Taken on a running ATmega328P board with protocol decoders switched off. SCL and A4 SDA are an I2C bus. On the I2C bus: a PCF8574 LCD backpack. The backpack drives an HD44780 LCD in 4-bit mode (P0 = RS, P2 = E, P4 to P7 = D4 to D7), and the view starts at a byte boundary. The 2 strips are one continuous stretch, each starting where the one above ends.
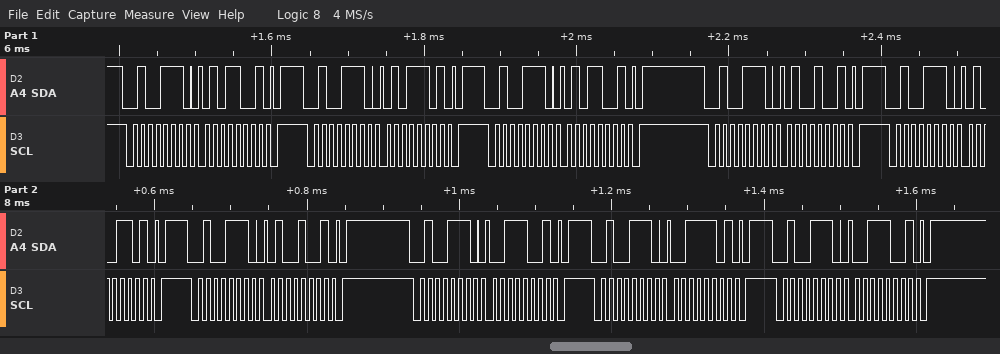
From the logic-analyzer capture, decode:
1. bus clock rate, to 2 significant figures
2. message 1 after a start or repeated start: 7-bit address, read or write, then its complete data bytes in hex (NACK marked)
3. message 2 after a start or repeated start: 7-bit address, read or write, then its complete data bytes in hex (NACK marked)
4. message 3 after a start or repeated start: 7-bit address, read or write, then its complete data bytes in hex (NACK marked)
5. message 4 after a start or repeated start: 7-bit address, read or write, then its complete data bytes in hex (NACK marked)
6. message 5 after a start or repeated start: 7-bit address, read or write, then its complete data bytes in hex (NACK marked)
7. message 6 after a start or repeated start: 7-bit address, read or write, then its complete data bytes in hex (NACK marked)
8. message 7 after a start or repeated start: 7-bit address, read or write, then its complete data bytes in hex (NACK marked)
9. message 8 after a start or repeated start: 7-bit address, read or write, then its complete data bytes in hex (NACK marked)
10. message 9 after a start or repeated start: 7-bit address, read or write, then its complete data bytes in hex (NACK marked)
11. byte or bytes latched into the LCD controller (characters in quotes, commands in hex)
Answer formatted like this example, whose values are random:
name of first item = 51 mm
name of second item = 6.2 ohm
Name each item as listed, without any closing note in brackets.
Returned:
bus clock rate, to 2 significant figures = 100 kHz
message 1 after a start or repeated start: 7-bit address, read or write, then its complete data bytes in hex = 0x27 write: 59
message 2 after a start or repeated start: 7-bit address, read or write, then its complete data bytes in hex = 0x27 write: 5D
message 3 after a start or repeated start: 7-bit address, read or write, then its complete data bytes in hex = 0x27 write: 59
message 4 after a start or repeated start: 7-bit address, read or write, then its complete data bytes in hex = 0x27 write: 49
message 5 after a start or repeated start: 7-bit address, read or write, then its complete data bytes in hex = 0x27 write: 4D
message 6 after a start or repeated start: 7-bit address, read or write, then its complete data bytes in hex = 0x27 write: 49
message 7 after a start or repeated start: 7-bit address, read or write, then its complete data bytes in hex = 0x27 write: 39
message 8 after a start or repeated start: 7-bit address, read or write, then its complete data bytes in hex = 0x27 write: 3D
message 9 after a start or repeated start: 7-bit address, read or write, then its complete data bytes in hex = 0x27 write: 39
byte or bytes latched into the LCD controller = 'T'
